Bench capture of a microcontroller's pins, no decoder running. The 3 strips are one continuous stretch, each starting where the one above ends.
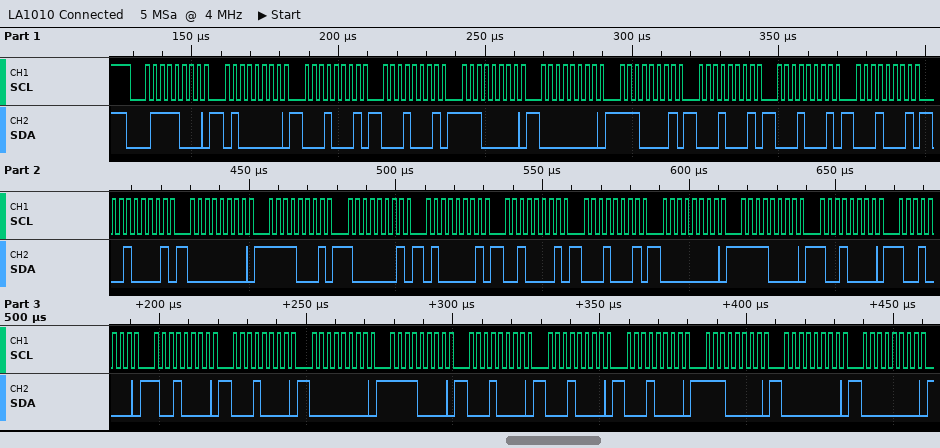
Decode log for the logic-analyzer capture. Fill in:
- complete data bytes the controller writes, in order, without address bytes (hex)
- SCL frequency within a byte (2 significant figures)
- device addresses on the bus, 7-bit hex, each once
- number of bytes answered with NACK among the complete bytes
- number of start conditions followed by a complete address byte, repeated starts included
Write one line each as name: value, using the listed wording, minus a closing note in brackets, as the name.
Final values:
complete data bytes the controller writes, in order, without address bytes: 40 11 11 E0 00 E1 11 11 11 21 00 F1 81 41 21 11 00 F0 90 90 90 10 00 F0 10 10 10 E0 00 00
SCL frequency within a byte: 400 kHz
device addresses on the bus, 7-bit hex, each once: 0x3C
number of bytes answered with NACK among the complete bytes: 0
number of start conditions followed by a complete address byte, repeated starts included: 1
